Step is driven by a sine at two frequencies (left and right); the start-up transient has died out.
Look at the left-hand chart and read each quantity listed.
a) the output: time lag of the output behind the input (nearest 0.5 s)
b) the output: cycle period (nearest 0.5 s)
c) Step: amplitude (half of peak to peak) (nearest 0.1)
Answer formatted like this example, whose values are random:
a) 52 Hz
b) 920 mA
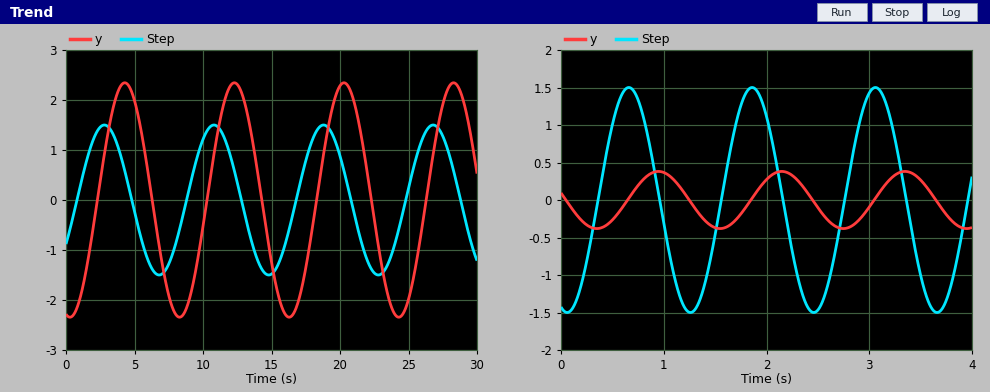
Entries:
a) 1.5 s
b) 8.0 s
c) 1.5
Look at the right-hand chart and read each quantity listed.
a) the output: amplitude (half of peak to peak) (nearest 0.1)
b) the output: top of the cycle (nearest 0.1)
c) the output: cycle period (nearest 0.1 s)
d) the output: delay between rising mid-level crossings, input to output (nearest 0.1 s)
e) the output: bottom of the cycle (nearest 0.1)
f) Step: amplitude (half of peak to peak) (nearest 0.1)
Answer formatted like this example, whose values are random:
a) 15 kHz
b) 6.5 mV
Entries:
a) 0.4
b) 0.4
c) 1.2 s
d) 0.3 s
e) -0.4
f) 1.5
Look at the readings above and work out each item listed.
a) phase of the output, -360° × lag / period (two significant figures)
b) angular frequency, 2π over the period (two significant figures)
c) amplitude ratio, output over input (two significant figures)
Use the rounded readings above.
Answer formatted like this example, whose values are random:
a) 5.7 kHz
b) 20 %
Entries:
a) -90°
b) 5.2 rad/s
c) 0.27
